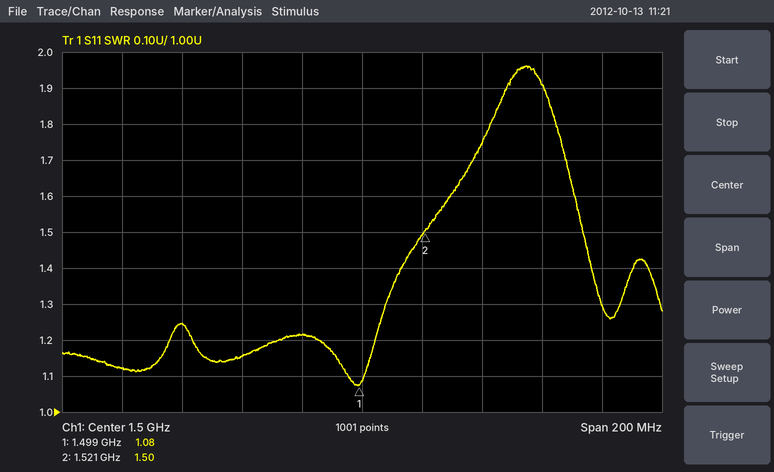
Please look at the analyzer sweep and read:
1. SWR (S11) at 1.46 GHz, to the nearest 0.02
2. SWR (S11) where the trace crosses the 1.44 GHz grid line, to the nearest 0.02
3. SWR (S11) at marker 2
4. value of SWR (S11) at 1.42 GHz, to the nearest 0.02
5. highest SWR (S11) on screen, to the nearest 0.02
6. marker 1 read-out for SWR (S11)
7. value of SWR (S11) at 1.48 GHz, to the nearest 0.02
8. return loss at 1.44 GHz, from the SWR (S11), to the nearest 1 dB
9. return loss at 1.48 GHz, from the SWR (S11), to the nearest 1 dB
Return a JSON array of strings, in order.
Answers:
["1.16", "1.24", "1.50", "1.12", "1.96", "1.08", "1.22", "19 dB", "20 dB"]
